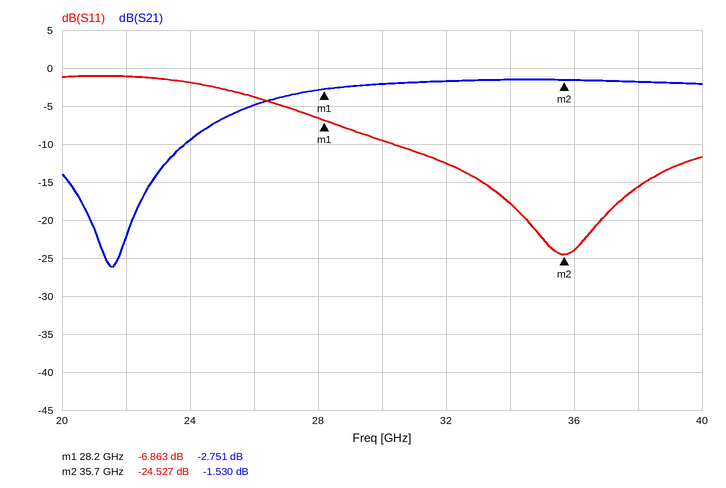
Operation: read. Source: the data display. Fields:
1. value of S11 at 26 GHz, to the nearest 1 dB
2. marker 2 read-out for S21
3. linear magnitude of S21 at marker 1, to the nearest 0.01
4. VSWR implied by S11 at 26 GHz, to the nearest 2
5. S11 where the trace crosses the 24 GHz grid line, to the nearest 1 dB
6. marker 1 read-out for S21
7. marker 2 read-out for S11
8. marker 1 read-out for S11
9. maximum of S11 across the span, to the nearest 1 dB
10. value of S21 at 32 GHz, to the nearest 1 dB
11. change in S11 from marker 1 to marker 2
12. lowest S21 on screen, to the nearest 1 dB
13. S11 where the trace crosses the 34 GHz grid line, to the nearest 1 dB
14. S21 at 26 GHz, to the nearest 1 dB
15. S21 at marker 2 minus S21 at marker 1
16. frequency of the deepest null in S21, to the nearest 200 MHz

-4 dB
-1.530 dB
0.73
4
-2 dB
-2.751 dB
-24.527 dB
-6.863 dB
-1 dB
-2 dB
-17.664 dB
-26 dB
-18 dB
-5 dB
1.221 dB
21.6 GHz
